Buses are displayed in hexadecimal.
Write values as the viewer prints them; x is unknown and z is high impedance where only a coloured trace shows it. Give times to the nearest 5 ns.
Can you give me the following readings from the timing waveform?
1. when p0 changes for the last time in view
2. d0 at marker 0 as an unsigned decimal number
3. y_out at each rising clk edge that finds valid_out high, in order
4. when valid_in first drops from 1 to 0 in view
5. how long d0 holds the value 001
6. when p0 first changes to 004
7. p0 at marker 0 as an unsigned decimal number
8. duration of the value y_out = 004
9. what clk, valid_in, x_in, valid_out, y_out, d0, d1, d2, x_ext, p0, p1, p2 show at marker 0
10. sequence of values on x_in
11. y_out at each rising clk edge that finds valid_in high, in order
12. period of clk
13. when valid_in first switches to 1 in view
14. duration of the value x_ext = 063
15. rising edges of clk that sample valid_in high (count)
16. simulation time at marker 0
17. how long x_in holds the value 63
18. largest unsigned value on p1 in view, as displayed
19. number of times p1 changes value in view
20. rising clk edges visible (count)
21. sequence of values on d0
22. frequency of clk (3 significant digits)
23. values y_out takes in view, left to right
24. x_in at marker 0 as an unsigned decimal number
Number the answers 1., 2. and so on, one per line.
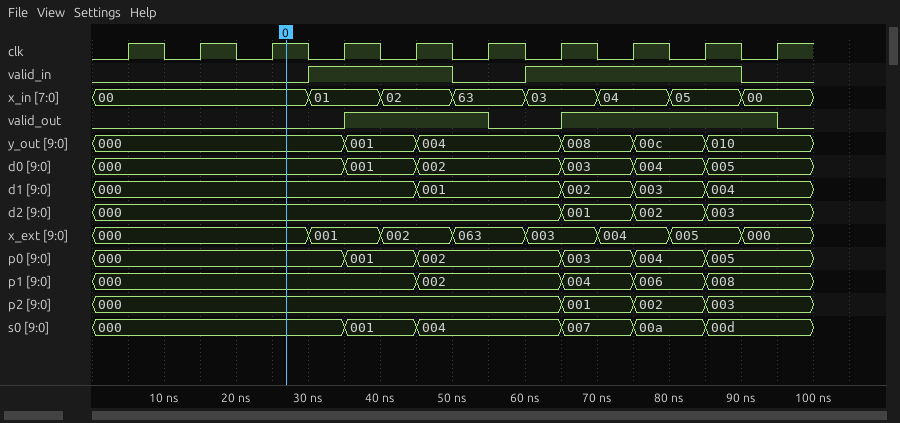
1. 85 ns
2. 0
3. 001, 004, 008, 00c, 010
4. 50 ns
5. 10 ns
6. 75 ns
7. 0
8. 20 ns
9. clk=1, valid_in=0, x_in=00, valid_out=0, y_out=000, d0=000, d1=000, d2=000, x_ext=000, p0=000, p1=000, p2=000
10. 00, 01, 02, 63, 03, 04, 05, 00
11. 000, 001, 004, 008, 00c
12. 10 ns
13. 30 ns
14. 10 ns
15. 5
16. 25 ns
17. 10 ns
18. 008
19. 4
20. 10
21. 000, 001, 002, 003, 004, 005
22. 100 MHz
23. 000, 001, 004, 008, 00c, 010
24. 0
